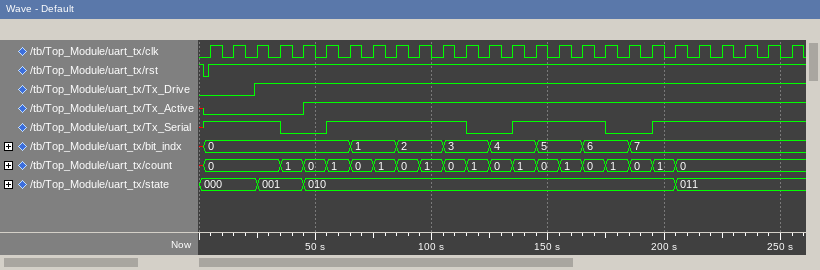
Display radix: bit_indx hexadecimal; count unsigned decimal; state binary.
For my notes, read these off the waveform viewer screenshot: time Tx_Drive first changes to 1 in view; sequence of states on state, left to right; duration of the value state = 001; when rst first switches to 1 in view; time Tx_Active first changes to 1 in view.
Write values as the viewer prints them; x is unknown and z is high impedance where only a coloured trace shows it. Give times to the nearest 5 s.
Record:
25 s
000, 001, 010, 011
20 s
5 s
45 s
